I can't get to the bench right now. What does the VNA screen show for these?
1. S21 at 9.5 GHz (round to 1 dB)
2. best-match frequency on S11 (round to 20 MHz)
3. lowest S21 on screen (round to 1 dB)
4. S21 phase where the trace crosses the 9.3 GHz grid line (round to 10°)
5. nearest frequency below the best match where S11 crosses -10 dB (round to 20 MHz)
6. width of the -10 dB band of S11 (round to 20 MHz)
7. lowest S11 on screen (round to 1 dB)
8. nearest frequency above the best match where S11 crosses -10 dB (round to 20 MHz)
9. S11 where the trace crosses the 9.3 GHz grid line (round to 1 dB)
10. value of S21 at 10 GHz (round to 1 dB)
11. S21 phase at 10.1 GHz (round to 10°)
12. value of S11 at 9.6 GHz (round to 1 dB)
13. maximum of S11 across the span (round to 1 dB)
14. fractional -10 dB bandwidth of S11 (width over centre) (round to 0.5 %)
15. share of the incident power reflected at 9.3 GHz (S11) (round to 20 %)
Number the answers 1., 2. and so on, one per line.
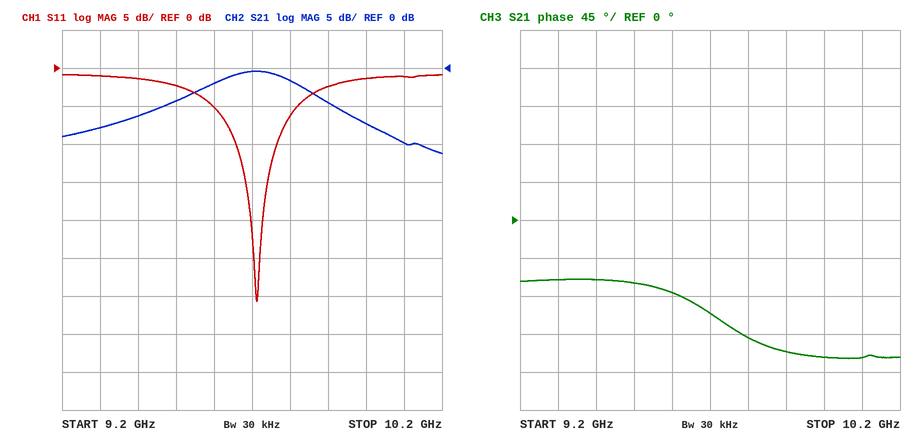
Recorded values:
1. -4 dB
2. 9.72 GHz
3. -11 dB
4. -70°
5. 9.66 GHz
6. 100 MHz
7. -31 dB
8. 9.76 GHz
9. -1 dB
10. -7 dB
11. -160°
12. -5 dB
13. -1 dB
14. 1.0 %
15. 80 %
